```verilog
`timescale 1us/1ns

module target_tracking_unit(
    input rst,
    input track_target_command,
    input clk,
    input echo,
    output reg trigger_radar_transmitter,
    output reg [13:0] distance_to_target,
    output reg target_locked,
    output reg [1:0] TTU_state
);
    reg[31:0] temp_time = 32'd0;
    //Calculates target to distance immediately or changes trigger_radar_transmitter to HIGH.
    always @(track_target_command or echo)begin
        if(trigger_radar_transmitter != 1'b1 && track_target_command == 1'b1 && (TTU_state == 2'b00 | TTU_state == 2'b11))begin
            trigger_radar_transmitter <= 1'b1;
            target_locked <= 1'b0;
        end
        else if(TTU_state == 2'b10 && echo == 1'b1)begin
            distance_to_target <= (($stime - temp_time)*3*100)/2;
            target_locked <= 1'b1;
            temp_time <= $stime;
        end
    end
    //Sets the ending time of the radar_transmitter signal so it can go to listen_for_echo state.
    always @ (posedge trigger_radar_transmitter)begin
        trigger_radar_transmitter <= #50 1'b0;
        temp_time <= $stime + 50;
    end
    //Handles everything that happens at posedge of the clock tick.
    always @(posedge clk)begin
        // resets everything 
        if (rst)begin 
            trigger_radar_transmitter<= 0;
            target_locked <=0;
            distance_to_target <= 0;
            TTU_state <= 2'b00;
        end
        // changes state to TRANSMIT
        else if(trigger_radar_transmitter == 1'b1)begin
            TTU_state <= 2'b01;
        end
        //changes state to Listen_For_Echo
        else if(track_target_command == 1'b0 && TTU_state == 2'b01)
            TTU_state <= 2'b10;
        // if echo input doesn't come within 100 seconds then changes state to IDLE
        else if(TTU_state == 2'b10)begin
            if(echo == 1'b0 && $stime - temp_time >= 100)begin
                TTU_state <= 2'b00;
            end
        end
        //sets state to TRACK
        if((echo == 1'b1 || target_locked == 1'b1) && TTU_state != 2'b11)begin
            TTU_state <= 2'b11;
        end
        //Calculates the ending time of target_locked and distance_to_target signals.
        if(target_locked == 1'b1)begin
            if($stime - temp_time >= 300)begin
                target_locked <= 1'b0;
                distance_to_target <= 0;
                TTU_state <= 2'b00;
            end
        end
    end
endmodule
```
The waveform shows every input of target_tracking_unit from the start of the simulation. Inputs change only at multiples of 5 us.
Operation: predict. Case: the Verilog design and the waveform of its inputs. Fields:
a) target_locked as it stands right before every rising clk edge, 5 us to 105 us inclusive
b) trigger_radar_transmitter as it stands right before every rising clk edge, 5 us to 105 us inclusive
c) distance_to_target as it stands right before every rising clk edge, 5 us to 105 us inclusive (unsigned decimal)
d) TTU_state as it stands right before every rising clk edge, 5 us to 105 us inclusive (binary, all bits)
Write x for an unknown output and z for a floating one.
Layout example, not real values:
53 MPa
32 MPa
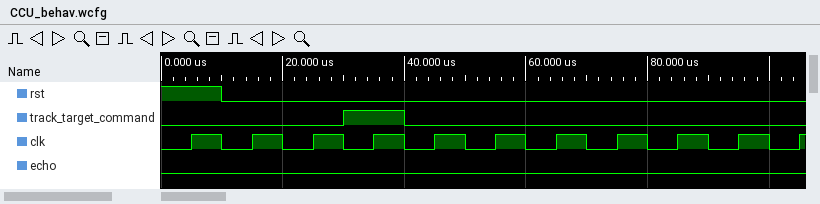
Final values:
x 0 0 0 0 0 0 0 0 0 0
x 0 0 1 1 1 1 1 0 0 0
x, 0, 0, 0, 0, 0, 0, 0, 0, 0, 0
x, 00, 00, 00, 01, 01, 01, 01, 01, 10, 10
